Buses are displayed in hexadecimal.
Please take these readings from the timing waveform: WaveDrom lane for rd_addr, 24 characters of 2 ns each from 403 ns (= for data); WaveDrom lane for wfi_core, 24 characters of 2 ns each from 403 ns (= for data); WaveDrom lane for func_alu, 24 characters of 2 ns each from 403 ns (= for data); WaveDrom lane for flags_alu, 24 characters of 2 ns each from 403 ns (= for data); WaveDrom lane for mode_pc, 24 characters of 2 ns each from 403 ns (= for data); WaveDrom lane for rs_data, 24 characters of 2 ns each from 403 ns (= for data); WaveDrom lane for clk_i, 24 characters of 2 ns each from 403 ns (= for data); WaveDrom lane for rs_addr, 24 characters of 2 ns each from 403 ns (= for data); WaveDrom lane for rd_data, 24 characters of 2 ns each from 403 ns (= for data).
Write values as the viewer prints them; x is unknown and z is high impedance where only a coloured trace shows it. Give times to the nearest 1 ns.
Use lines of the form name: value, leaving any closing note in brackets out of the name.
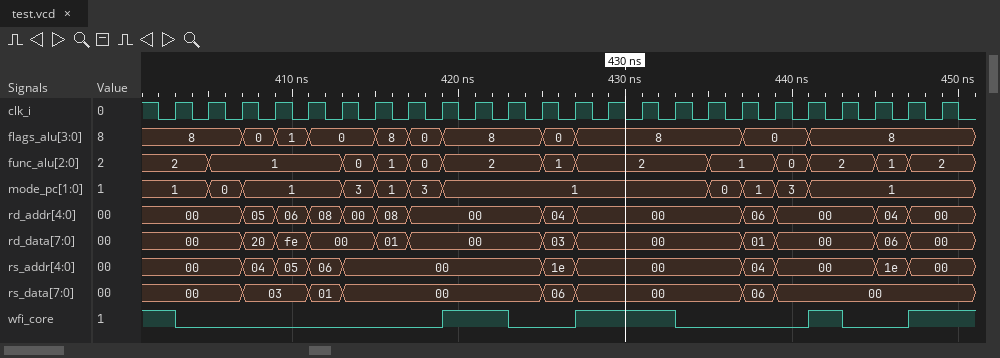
WaveDrom lane for rd_addr, 24 characters of 2 ns each from 403 ns: {name: 'rd_addr', wave: '=.======...==....==..==.', data: '00 05 06 08 00 08 00 04 00 06 00 04 00'}
WaveDrom lane for wfi_core, 24 characters of 2 ns each from 403 ns: {name: 'wfi_core', wave: '0.......1.0.1..0...10.1.'}
WaveDrom lane for func_alu, 24 characters of 2 ns each from 403 ns: {name: 'func_alu', wave: '==...====..==...=.==.==.', data: '2 1 0 1 0 2 1 2 1 0 2 1 2'}
WaveDrom lane for flags_alu, 24 characters of 2 ns each from 403 ns: {name: 'flags_alu', wave: '=.===.===..==....=.=....', data: '8 0 1 0 8 0 8 0 8 0 8'}
WaveDrom lane for mode_pc, 24 characters of 2 ns each from 403 ns: {name: 'mode_pc', wave: '===..====.......====....', data: '1 0 1 3 1 3 1 0 1 3 1'}
WaveDrom lane for rs_data, 24 characters of 2 ns each from 403 ns: {name: 'rs_data', wave: '=.=.==.....==....==.....', data: '00 03 01 00 06 00 06 00'}
WaveDrom lane for clk_i, 24 characters of 2 ns each from 403 ns: {name: 'clk_i', wave: 'p.......................'}
WaveDrom lane for rs_addr, 24 characters of 2 ns each from 403 ns: {name: 'rs_addr', wave: '=.====.....==....==..==.', data: '00 04 05 06 00 1e 00 04 00 1e 00'}
WaveDrom lane for rd_data, 24 characters of 2 ns each from 403 ns: {name: 'rd_data', wave: '=.===.==...==....==..==.', data: '00 20 fe 00 01 00 03 00 01 00 06 00'}
